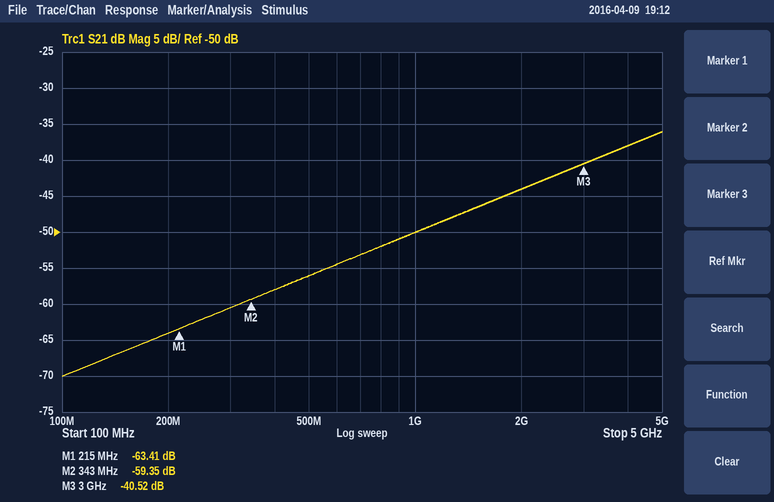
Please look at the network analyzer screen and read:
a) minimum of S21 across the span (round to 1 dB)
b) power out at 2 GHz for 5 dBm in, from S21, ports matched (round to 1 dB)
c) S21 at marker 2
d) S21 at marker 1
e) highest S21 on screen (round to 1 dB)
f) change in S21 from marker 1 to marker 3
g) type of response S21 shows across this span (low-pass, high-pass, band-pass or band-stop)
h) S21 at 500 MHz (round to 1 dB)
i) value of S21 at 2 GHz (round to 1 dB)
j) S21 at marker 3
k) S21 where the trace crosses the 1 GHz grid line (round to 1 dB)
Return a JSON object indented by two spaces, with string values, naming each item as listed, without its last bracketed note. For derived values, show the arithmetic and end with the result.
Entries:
{
  "minimum of S21 across the span": "-70 dB",
  "power out at 2 GHz for 5 dBm in, from S21, ports matched": "5 dBm + (-44 dB) = -39 dBm",
  "S21 at marker 2": "-59.35 dB",
  "S21 at marker 1": "-63.41 dB",
  "highest S21 on screen": "-36 dB",
  "change in S21 from marker 1 to marker 3": "-40.52 − (-63.41) = 22.89 dB",
  "type of response S21 shows across this span": "high-pass",
  "S21 at 500 MHz": "-56 dB",
  "value of S21 at 2 GHz": "-44 dB",
  "S21 at marker 3": "-40.52 dB",
  "S21 where the trace crosses the 1 GHz grid line": "-50 dB"
}
